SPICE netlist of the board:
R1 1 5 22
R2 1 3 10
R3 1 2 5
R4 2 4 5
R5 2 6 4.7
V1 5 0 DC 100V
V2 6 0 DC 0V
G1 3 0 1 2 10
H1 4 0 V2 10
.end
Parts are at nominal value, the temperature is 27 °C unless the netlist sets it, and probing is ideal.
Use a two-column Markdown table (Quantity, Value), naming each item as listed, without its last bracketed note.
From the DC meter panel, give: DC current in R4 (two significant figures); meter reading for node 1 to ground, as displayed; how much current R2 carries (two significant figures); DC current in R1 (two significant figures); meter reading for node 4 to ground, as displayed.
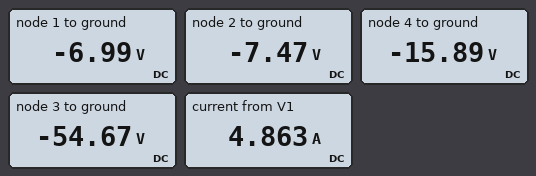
| Quantity | Value |
|---|---|
| DC current in R4 | 1.7 A |
| meter reading for node 1 to ground, as displayed | -6.99 V |
| how much current R2 carries | 4.8 A |
| DC current in R1 | 4.9 A |
| meter reading for node 4 to ground, as displayed | -15.89 V |
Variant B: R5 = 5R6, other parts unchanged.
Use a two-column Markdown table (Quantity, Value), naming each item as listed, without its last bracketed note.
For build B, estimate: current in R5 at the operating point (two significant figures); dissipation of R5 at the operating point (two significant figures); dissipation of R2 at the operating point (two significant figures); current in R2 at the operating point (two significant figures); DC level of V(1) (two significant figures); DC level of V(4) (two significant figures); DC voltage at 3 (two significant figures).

| Quantity | Value |
|---|---|
| current in R5 at the operating point | 710 mA |
| dissipation of R5 at the operating point | 2.8 W |
| dissipation of R2 at the operating point | 180 W |
| current in R2 at the operating point | 4.3 A |
| DC level of V(1) | 4.4 V |
| DC level of V(4) | 7.1 V |
| DC voltage at 3 | -38 V |
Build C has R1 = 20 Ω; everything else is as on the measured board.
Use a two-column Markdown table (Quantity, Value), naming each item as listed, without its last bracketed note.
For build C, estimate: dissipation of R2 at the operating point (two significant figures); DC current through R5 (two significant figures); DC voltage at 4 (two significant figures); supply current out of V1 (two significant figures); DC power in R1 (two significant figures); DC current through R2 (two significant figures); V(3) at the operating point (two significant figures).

| Quantity | Value |
|---|---|
| dissipation of R2 at the operating point | 280 W |
| DC current through R5 | 1.8 A |
| DC voltage at 4 | -18 V |
| supply current out of V1 | 5.4 A |
| DC power in R1 | 580 W |
| DC current through R2 | 5.3 A |
| V(3) at the operating point | -61 V |
